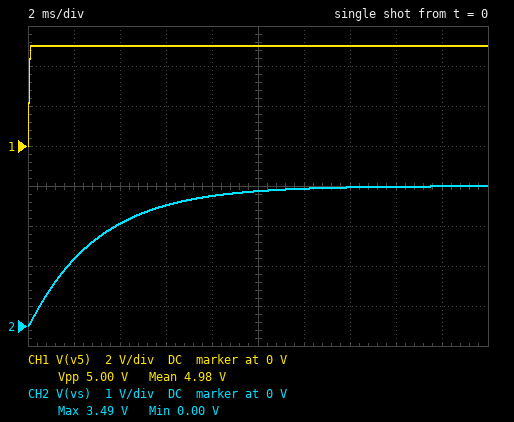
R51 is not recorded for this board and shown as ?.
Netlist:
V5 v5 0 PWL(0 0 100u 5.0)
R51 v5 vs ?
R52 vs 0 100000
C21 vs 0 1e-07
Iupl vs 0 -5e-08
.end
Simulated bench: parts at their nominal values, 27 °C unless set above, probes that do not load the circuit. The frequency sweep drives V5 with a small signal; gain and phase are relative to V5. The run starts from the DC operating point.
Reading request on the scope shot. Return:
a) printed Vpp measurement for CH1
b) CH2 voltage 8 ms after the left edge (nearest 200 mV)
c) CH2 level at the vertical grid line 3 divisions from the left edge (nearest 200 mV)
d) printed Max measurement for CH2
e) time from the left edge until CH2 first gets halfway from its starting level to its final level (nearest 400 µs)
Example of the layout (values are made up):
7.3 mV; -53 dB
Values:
5.00 V; 3.2 V; 3.0 V; 3.49 V; 2.0 ms
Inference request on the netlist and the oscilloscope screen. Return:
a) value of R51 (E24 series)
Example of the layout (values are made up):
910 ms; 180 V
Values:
43 kΩ
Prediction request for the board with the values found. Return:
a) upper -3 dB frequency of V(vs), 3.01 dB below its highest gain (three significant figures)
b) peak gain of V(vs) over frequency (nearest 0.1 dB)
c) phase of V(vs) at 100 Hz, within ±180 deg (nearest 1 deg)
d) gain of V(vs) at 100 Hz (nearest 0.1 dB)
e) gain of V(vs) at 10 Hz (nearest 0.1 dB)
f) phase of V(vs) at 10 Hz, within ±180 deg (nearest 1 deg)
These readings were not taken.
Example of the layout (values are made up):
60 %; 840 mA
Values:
52.9 Hz; -3.1 dB; -62 deg; -9.7 dB; -3.3 dB; -11 deg
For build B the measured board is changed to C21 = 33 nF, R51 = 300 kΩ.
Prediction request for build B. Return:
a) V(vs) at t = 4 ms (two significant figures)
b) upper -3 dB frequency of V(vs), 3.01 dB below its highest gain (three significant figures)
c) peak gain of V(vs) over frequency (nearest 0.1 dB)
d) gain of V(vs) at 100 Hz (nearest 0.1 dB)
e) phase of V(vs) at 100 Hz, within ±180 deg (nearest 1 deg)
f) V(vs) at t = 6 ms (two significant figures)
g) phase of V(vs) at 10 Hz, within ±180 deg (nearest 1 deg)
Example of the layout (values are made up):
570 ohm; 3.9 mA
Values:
1.0 V; 64.3 Hz; -12.0 dB; -17.4 dB; -57 deg; 1.1 V; -9 deg
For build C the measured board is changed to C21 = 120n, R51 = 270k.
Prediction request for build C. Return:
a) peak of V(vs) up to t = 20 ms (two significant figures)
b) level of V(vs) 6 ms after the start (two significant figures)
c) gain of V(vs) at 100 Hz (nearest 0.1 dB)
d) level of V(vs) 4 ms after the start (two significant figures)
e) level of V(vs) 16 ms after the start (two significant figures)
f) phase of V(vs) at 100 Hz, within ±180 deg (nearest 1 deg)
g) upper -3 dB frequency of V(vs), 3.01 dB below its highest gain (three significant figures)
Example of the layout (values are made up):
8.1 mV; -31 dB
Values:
1.2 V; 670 mV; -26.3 dB; 490 mV; 1.1 V; -80 deg; 18.2 Hz
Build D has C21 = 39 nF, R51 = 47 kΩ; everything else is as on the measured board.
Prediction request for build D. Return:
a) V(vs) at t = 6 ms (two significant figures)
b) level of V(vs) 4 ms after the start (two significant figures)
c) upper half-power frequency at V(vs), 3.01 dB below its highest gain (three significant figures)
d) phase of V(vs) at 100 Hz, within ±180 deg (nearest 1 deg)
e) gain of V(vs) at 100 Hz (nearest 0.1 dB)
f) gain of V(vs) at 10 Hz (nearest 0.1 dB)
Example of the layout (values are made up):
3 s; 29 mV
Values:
3.4 V; 3.3 V; 128 Hz; -38 deg; -5.4 dB; -3.4 dB
